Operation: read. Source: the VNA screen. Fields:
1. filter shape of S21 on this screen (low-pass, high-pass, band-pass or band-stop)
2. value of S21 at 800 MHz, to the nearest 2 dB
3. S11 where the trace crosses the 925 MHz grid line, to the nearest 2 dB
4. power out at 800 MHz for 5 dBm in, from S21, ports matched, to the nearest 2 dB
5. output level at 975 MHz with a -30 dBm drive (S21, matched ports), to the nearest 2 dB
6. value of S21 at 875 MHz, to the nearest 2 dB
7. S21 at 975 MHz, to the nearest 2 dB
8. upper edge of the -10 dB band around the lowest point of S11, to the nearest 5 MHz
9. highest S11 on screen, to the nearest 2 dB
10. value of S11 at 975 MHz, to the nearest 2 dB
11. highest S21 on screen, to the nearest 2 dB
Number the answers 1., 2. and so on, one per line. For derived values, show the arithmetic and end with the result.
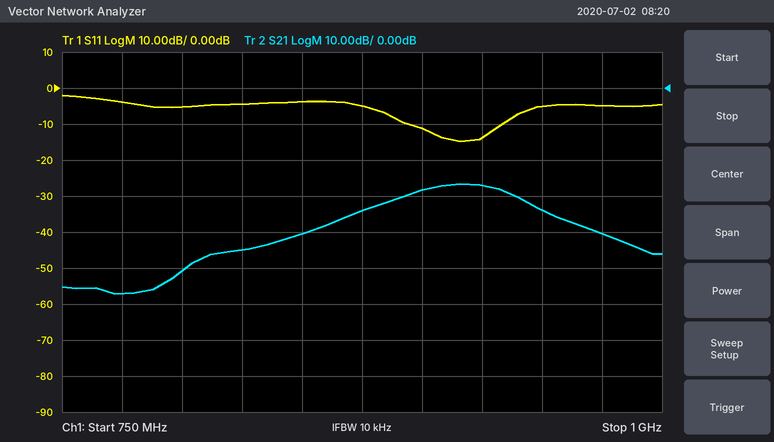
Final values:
1. band-pass
2. -50 dB
3. -14 dB
4. 5 dBm + (-50 dB) = -46 dBm
5. -30 dBm + (-40 dB) = -70 dBm
6. -34 dB
7. -40 dB
8. 935 MHz
9. -2 dB
10. -4 dB
11. -26 dB
